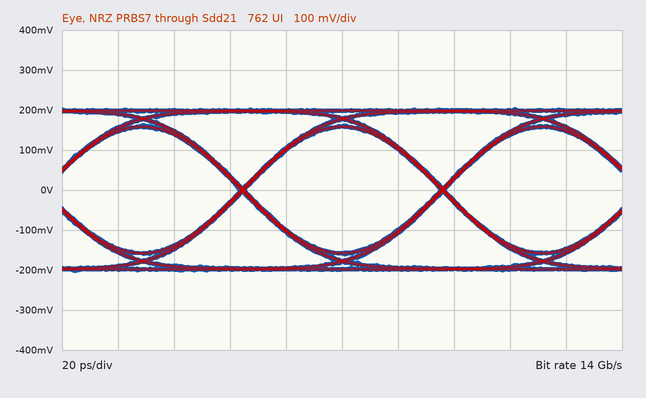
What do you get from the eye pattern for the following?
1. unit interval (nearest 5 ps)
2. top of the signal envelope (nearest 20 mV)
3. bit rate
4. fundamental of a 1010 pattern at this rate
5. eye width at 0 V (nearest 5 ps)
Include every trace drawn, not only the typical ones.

70 ps
200 mV
14 Gb/s
7 GHz
70 ps
